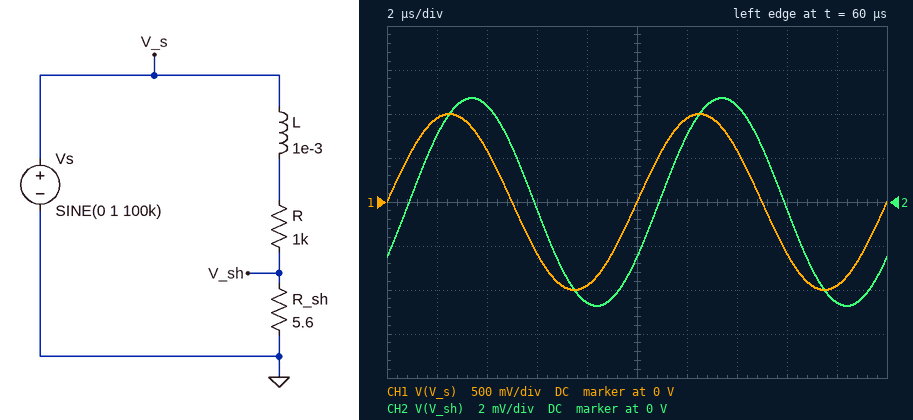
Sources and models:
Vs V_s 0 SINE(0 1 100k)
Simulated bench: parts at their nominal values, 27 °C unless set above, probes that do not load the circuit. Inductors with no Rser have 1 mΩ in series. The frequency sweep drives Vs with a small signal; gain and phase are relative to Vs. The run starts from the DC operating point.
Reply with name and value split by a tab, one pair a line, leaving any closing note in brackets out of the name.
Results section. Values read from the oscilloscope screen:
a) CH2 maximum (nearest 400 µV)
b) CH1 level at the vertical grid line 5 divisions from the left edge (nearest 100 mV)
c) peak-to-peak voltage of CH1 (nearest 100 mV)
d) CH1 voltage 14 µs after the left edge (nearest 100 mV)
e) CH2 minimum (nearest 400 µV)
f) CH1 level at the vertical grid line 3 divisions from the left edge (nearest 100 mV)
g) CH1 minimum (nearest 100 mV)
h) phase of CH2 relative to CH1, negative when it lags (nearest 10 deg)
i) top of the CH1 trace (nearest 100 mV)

CH2 maximum	4.8 mV
CH1 level at the vertical grid line 5 divisions from the left edge	0 V
peak-to-peak voltage of CH1	2.0 V
CH1 voltage 14 µs after the left edge	600 mV
CH2 minimum	-4.8 mV
CH1 level at the vertical grid line 3 divisions from the left edge	-600 mV
CH1 minimum	-1.0 V
phase of CH2 relative to CH1, negative when it lags	-30 deg
top of the CH1 trace	1.0 V
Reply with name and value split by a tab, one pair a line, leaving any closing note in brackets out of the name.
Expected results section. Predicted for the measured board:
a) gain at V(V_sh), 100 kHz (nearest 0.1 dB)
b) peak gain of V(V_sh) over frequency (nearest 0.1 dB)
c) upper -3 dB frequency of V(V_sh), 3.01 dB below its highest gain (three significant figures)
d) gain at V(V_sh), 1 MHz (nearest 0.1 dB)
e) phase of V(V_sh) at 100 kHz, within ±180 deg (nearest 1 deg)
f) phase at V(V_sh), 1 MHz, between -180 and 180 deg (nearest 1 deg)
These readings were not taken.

gain at V(V_sh), 100 kHz	-46.5 dB
peak gain of V(V_sh) over frequency	-45.1 dB
upper -3 dB frequency of V(V_sh), 3.01 dB below its highest gain	160 kHz
gain at V(V_sh), 1 MHz	-61.1 dB
phase of V(V_sh) at 100 kHz, within ±180 deg	-32 deg
phase at V(V_sh), 1 MHz, between -180 and 180 deg	-81 deg
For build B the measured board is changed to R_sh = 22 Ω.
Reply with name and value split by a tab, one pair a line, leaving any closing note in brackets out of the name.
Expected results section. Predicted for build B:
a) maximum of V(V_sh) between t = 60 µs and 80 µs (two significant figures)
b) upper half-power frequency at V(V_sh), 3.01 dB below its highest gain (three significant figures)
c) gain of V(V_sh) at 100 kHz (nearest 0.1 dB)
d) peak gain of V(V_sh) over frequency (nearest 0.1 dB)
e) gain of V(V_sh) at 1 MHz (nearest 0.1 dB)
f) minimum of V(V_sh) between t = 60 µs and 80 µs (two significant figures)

maximum of V(V_sh) between t = 60 µs and 80 µs	18 mV
upper half-power frequency at V(V_sh), 3.01 dB below its highest gain	163 kHz
gain of V(V_sh) at 100 kHz	-34.7 dB
peak gain of V(V_sh) over frequency	-33.3 dB
gain of V(V_sh) at 1 MHz	-49.2 dB
minimum of V(V_sh) between t = 60 µs and 80 µs	-18 mV
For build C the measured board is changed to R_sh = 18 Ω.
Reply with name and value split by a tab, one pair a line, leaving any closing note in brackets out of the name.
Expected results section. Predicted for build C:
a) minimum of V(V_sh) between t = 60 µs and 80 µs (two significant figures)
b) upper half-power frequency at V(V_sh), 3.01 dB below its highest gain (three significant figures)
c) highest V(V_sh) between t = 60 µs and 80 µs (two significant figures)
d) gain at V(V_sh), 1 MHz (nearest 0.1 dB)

minimum of V(V_sh) between t = 60 µs and 80 µs	-15 mV
upper half-power frequency at V(V_sh), 3.01 dB below its highest gain	162 kHz
highest V(V_sh) between t = 60 µs and 80 µs	15 mV
gain at V(V_sh), 1 MHz	-51.0 dB
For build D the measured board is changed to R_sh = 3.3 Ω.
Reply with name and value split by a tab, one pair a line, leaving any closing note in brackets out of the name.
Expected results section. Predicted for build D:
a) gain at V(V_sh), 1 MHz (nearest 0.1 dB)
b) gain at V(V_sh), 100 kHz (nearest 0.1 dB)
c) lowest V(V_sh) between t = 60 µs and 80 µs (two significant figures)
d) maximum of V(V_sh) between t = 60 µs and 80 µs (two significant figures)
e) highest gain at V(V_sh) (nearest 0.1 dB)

gain at V(V_sh), 1 MHz	-65.7 dB
gain at V(V_sh), 100 kHz	-51.1 dB
lowest V(V_sh) between t = 60 µs and 80 µs	-2.8 mV
maximum of V(V_sh) between t = 60 µs and 80 µs	2.8 mV
highest gain at V(V_sh)	-49.7 dB
